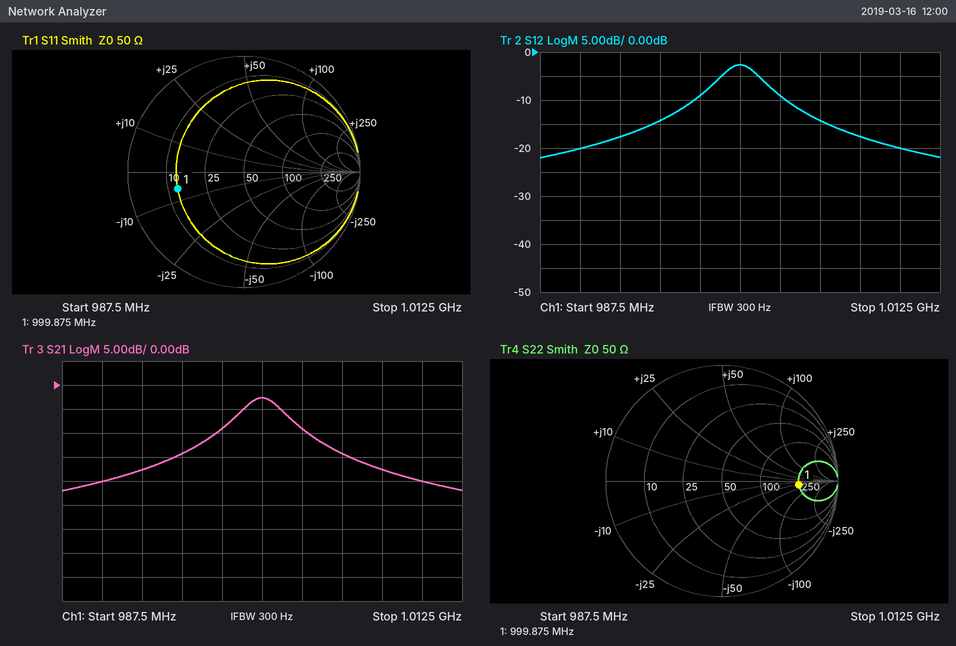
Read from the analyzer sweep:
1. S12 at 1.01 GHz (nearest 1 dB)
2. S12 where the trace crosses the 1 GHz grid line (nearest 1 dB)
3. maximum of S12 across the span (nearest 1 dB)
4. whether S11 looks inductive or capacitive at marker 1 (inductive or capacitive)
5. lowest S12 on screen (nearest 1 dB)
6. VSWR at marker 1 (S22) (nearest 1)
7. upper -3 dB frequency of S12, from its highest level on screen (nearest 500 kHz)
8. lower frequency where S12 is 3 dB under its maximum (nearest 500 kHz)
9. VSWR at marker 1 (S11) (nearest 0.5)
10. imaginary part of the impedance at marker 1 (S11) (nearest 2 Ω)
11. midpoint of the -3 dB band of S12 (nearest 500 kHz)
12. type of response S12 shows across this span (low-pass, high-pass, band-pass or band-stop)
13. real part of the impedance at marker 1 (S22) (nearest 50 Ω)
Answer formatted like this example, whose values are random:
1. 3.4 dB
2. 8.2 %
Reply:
1. -20 dB
2. -3 dB
3. -3 dB
4. capacitive
5. -22 dB
6. 5
7. 1.0015 GHz
8. 998.5 MHz
9. 4.0
10. -6 Ω
11. 1.0000 GHz
12. band-pass
13. 250 Ω
